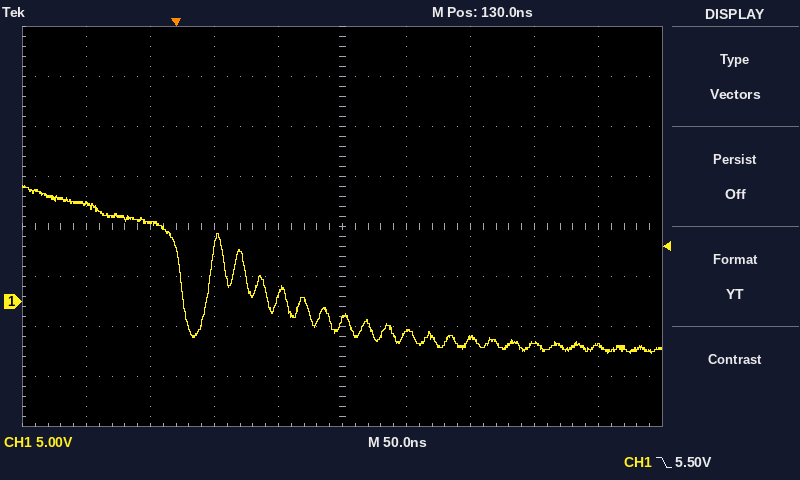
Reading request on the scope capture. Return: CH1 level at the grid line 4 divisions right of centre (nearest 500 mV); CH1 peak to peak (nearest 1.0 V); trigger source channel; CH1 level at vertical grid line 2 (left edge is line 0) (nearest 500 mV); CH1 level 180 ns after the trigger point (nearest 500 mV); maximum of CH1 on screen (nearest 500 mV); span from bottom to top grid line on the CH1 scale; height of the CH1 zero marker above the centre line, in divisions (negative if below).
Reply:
-4.5 V
17.0 V
CH1
8.0 V
-3.0 V
11.5 V
40 V
-1.5 div
